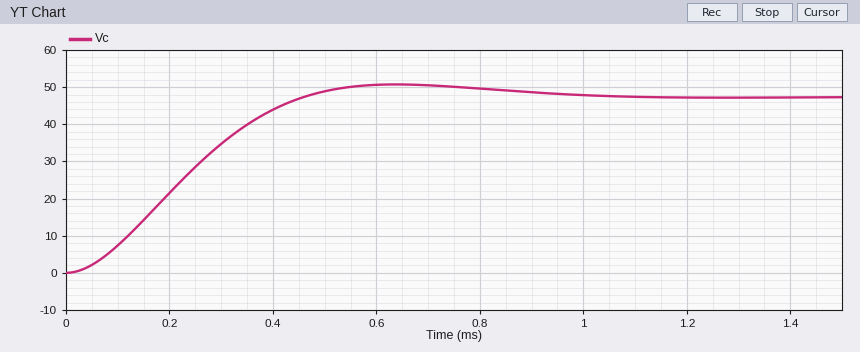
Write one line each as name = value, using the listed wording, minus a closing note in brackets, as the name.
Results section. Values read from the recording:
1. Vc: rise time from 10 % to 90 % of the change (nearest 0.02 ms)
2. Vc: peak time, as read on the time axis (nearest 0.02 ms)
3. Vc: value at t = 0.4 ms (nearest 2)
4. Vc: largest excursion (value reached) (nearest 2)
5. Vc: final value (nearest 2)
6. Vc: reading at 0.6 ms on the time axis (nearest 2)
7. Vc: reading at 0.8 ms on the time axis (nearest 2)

Vc: rise time from 10 % to 90 % of the change = 0.30 ms
Vc: peak time, as read on the time axis = 0.64 ms
Vc: value at t = 0.4 ms = 44
Vc: largest excursion (value reached) = 50
Vc: final value = 48
Vc: reading at 0.6 ms on the time axis = 50
Vc: reading at 0.8 ms on the time axis = 50
